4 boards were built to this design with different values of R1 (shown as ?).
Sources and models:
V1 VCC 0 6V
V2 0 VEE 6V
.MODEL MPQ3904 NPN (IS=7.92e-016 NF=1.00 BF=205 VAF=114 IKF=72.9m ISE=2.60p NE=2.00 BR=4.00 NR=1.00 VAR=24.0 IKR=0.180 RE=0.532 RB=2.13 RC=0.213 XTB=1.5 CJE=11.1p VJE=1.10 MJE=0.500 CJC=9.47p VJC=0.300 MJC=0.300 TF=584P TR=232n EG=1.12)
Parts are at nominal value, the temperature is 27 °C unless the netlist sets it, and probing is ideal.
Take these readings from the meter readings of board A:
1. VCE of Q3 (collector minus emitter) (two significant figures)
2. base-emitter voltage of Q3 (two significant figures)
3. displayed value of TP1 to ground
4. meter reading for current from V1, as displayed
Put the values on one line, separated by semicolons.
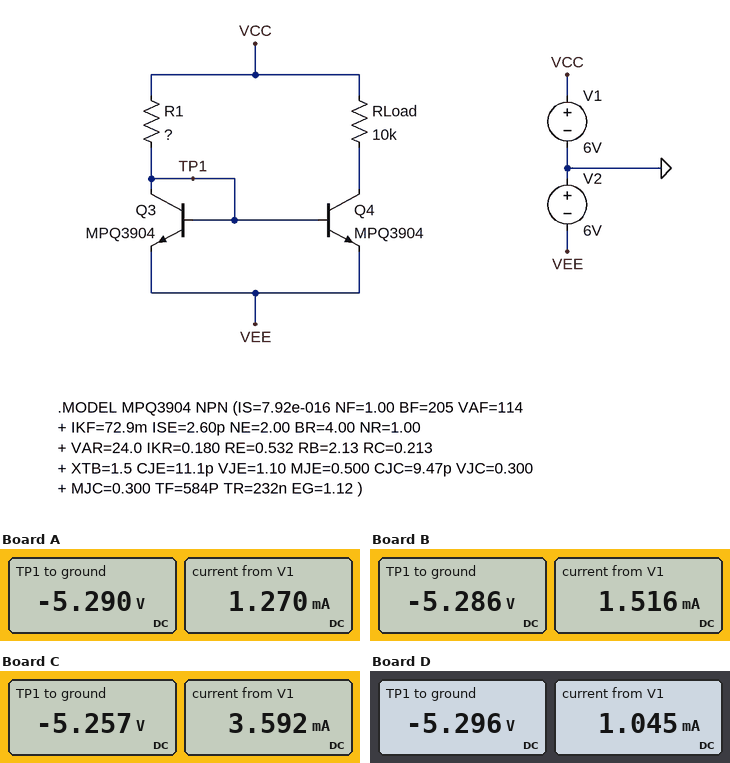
710 mV; 710 mV; -5.290 V; 1.270 mA
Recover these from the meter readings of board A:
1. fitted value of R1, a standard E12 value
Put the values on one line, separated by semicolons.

18 kΩ
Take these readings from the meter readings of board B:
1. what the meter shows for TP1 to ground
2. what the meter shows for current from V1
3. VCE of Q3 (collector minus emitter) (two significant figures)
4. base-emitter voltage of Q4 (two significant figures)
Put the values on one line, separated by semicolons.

-5.286 V; 1.516 mA; 710 mV; 710 mV
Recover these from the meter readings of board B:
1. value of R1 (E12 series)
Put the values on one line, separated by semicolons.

15 kΩ
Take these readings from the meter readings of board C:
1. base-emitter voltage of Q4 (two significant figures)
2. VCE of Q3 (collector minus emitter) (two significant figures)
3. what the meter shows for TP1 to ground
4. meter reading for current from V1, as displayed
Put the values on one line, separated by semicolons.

740 mV; 740 mV; -5.257 V; 3.592 mA
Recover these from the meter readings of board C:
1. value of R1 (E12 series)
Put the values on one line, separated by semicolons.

4.7 kΩ
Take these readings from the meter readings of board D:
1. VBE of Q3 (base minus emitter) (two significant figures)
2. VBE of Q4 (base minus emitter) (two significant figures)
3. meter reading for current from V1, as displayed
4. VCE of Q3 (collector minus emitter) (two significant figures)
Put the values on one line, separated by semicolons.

700 mV; 700 mV; 1.045 mA; 700 mV
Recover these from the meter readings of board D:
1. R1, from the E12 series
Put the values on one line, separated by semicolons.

22 kΩ
